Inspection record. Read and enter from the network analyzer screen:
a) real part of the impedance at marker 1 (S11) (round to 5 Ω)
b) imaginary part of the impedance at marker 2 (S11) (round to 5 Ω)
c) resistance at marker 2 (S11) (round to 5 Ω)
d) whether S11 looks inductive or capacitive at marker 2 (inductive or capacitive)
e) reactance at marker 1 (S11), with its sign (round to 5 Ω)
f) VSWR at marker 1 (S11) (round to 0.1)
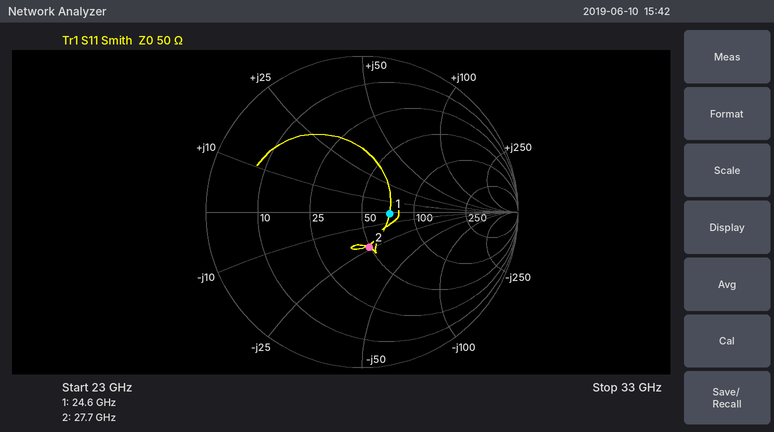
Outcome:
70 Ω
-25 Ω
50 Ω
capacitive
0 Ω
1.4
